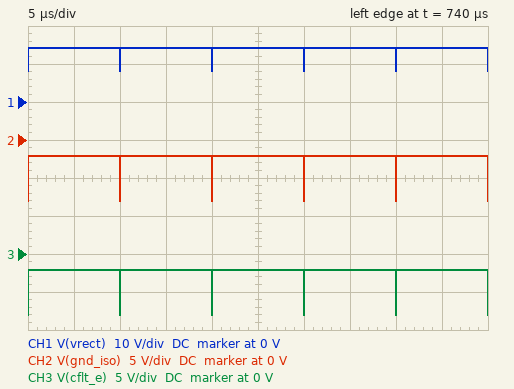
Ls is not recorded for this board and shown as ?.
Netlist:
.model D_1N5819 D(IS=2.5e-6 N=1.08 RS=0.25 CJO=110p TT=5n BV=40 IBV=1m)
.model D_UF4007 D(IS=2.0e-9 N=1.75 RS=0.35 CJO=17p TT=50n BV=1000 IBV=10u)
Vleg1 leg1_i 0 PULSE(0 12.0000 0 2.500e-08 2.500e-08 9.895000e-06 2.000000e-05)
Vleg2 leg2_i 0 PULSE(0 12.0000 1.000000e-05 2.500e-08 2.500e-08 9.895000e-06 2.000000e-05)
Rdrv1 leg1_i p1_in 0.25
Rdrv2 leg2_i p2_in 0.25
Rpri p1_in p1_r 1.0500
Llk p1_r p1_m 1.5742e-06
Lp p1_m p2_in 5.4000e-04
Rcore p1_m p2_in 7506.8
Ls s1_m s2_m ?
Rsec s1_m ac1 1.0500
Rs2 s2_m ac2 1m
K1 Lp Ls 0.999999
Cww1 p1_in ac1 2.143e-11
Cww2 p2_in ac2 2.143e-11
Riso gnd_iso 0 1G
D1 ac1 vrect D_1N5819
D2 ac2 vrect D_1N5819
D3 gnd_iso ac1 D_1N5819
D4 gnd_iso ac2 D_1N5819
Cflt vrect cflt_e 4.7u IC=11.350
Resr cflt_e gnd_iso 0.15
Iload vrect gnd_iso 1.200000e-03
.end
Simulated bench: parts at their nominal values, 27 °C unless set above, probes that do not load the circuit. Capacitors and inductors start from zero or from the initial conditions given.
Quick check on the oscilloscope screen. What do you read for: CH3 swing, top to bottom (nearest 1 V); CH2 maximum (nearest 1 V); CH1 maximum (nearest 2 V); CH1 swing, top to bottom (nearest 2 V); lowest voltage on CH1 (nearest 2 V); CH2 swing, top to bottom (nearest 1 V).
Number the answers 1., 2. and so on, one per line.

1. 6 V
2. -2 V
3. 14 V
4. 6 V
5. 8 V
6. 6 V
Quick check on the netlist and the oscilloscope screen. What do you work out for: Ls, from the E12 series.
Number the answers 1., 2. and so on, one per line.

1. 1 mH
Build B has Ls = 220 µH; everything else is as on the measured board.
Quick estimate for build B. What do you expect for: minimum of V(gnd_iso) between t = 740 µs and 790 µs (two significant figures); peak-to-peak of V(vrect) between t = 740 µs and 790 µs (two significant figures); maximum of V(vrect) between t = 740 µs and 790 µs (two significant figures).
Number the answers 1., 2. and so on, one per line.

1. -5.6 V
2. 6.0 V
3. 12 V
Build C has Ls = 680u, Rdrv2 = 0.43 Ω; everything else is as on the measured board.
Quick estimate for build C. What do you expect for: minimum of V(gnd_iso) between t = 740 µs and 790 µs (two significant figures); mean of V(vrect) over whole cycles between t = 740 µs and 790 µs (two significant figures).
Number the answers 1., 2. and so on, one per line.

1. -6.6 V
2. 13 V
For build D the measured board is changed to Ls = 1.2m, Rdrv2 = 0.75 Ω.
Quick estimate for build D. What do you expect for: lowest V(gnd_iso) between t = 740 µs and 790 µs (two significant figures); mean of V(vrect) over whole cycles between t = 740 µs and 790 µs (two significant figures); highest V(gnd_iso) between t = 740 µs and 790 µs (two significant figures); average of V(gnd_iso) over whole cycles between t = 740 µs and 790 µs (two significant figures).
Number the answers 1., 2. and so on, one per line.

1. -8.9 V
2. 15 V
3. -2.8 V
4. -2.9 V
